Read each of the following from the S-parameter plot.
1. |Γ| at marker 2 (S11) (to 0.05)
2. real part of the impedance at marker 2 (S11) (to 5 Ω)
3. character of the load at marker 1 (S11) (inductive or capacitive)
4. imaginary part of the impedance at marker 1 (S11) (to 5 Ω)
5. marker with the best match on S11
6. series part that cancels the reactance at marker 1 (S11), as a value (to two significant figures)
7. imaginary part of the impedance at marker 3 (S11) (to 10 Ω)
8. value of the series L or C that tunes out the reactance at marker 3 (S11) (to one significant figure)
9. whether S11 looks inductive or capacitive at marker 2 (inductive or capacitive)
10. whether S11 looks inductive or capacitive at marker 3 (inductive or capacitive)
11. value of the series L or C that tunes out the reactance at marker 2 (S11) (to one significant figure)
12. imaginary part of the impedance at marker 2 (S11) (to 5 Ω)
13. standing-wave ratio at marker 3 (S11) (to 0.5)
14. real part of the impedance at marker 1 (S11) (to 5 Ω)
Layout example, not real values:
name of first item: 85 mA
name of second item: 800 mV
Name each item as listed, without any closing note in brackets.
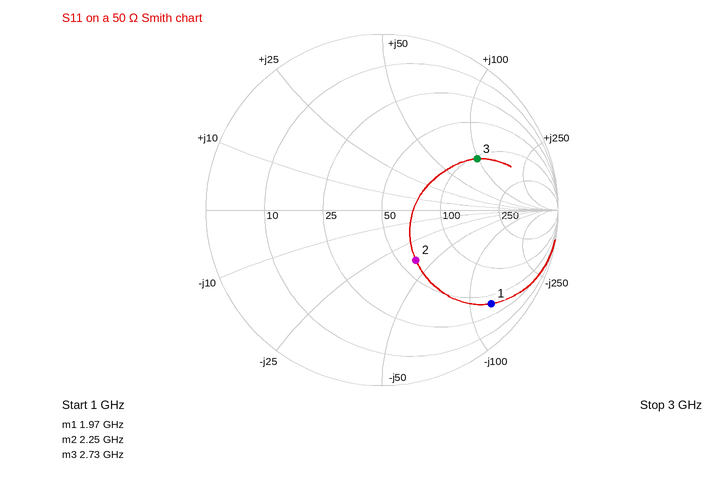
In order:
|Γ| at marker 2 (S11): 0.35
real part of the impedance at marker 2 (S11): 60 Ω
character of the load at marker 1 (S11): capacitive
imaginary part of the impedance at marker 1 (S11): -125 Ω
marker with the best match on S11: marker 2
series part that cancels the reactance at marker 1 (S11), as a value: 10 nH
imaginary part of the impedance at marker 3 (S11): +100 Ω
value of the series L or C that tunes out the reactance at marker 3 (S11): 600 fF
whether S11 looks inductive or capacitive at marker 2: capacitive
whether S11 looks inductive or capacitive at marker 3: inductive
value of the series L or C that tunes out the reactance at marker 2 (S11): 3 nH
imaginary part of the impedance at marker 2 (S11): -40 Ω
standing-wave ratio at marker 3 (S11): 4.0
real part of the impedance at marker 1 (S11): 40 Ω
